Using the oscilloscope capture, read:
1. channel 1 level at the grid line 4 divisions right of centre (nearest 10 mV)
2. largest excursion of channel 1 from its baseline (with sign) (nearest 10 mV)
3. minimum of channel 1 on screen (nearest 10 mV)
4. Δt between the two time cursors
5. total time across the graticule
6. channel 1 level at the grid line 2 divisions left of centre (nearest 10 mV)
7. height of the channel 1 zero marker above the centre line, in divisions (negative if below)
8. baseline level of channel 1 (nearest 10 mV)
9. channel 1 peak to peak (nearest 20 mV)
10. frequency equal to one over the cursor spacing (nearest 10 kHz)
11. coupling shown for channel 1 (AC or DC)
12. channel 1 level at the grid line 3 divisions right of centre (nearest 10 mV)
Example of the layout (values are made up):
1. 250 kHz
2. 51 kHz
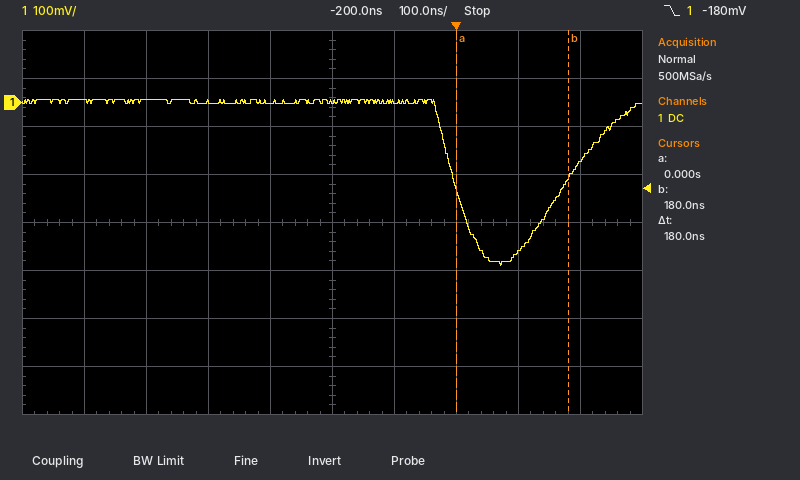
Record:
1. -120 mV
2. -340 mV
3. -340 mV
4. 180 ns
5. 1 µs
6. 0 mV
7. +2.5 div
8. 0 mV
9. 340 mV
10. 5.56 MHz
11. DC
12. -310 mV
